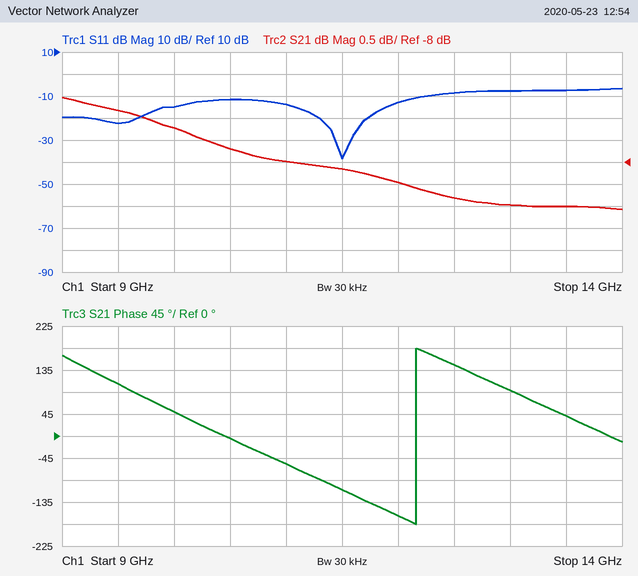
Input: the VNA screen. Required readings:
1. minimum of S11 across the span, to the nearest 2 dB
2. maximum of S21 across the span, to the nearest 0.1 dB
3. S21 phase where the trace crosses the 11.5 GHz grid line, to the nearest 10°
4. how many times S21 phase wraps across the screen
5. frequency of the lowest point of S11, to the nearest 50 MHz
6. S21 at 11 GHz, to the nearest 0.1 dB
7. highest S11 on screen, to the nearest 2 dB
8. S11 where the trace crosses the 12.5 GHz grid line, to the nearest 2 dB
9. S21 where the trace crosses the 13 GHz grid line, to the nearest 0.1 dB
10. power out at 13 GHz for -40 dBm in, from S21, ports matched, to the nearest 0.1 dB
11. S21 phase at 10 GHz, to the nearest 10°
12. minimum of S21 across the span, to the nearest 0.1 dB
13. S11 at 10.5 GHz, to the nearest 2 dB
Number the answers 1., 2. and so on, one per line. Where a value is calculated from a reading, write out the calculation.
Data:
1. -38 dB
2. -6.5 dB
3. -110°
4. 1
5. 11.50 GHz
6. -8.0 dB
7. -6 dB
8. -8 dB
9. -9.0 dB
10. -40 dBm + (-9.0 dB) = -49.0 dBm
11. 50°
12. -9.1 dB
13. -12 dB
